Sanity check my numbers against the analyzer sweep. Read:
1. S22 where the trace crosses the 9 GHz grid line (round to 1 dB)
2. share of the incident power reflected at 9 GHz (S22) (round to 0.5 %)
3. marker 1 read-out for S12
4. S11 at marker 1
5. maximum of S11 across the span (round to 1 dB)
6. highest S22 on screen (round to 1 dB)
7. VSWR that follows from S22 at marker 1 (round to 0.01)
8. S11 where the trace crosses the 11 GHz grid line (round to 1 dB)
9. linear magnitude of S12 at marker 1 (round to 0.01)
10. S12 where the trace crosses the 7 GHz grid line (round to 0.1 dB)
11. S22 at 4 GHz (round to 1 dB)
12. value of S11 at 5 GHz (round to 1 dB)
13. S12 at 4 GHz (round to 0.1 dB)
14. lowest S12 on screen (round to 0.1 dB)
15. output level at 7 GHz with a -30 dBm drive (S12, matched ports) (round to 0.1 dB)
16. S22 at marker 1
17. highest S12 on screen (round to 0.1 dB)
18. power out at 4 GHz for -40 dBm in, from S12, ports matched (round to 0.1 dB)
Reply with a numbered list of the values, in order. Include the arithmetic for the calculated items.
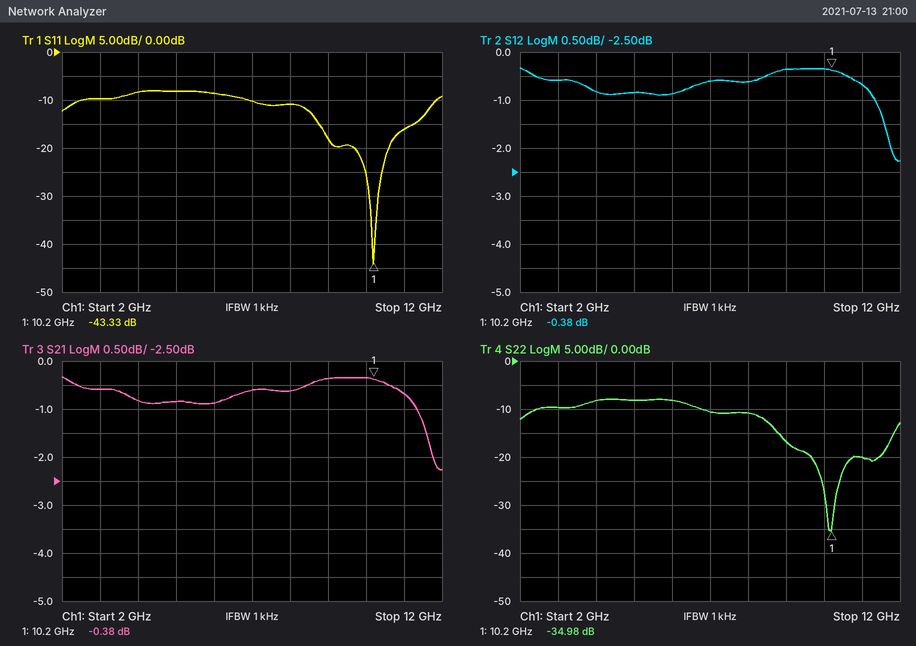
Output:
1. -17 dB
2. 10^(-17/10) ≈ 2.0 %
3. -0.38 dB
4. -43.33 dB
5. -8 dB
6. -8 dB
7. (1 + 0.0178)/(1 − 0.0178) ≈ 1.04
8. -16 dB
9. 10^(-0.38/20) ≈ 0.96
10. -0.6 dB
11. -8 dB
12. -8 dB
13. -0.8 dB
14. -2.3 dB
15. -30 dBm + (-0.6 dB) = -30.6 dBm
16. -34.98 dB
17. -0.3 dB
18. -40 dBm + (-0.8 dB) = -40.8 dBm
